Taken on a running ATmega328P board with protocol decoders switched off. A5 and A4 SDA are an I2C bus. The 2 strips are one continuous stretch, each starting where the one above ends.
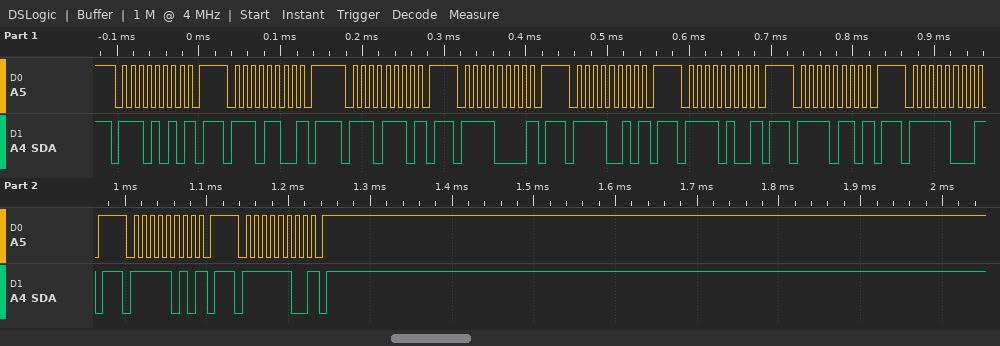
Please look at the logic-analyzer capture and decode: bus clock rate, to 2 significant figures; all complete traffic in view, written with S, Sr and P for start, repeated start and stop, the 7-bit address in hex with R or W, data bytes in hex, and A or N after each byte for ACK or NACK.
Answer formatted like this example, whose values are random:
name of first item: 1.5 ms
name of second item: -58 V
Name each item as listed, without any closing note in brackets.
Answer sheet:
bus clock rate, to 2 significant figures: 100 kHz
all complete traffic in view, written with S, Sr and P for start, repeated start and stop, the 7-bit address in hex with R or W, data bytes in hex, and A or N after each byte for ACK or NACK: S 75W N P S 76W N P S 77W N P S 78W N P S 79W N P S 7AW N P S 7BW N P S 7CW N P S 7DW N P S 7EW N P
